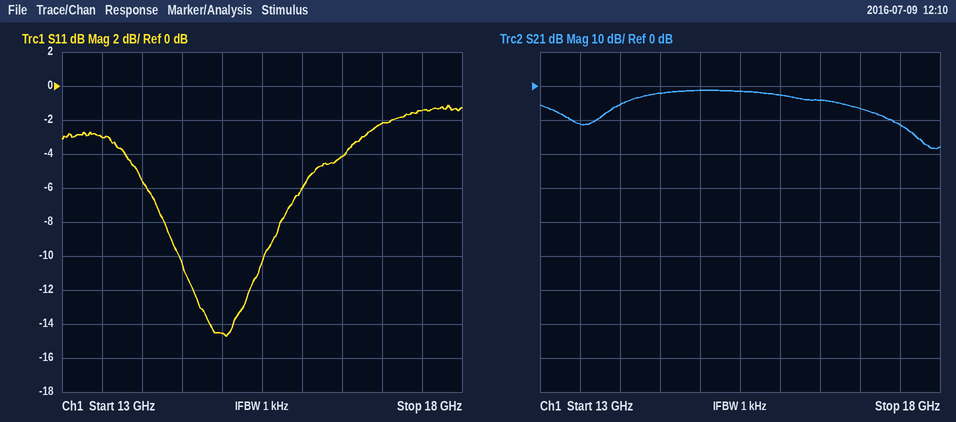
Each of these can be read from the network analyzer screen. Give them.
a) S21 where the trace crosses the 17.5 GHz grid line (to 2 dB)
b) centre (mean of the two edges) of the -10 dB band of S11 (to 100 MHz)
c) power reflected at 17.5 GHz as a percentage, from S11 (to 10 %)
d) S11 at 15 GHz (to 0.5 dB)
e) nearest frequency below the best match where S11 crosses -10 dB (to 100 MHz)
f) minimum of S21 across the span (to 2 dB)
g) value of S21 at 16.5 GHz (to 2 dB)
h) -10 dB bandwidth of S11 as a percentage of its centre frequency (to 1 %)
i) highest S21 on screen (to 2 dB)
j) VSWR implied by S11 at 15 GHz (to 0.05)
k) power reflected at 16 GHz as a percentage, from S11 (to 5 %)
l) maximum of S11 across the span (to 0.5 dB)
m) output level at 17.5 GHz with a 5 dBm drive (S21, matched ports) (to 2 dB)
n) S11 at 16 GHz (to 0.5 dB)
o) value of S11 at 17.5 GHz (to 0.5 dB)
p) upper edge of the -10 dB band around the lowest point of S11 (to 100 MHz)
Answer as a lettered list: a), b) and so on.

a) -12 dB
b) 15.0 GHz
c) 70 %
d) -14.5 dB
e) 14.5 GHz
f) -18 dB
g) -4 dB
h) 7 %
i) -2 dB
j) 1.45
k) 25 %
l) -1.0 dB
m) -6 dBm
n) -6.0 dB
o) -1.5 dB
p) 15.5 GHz
